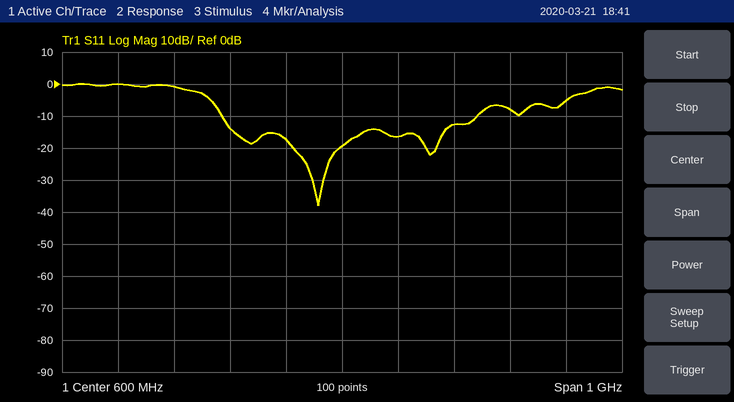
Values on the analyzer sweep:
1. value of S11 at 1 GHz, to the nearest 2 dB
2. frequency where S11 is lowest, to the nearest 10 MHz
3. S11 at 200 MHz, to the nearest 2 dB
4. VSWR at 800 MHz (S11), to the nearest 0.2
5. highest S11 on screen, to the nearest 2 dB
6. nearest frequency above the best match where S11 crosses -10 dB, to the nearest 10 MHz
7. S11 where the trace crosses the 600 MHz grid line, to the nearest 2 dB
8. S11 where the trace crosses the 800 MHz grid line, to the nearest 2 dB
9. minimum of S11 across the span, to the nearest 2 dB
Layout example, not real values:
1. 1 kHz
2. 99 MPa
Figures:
1. -6 dB
2. 560 MHz
3. 0 dB
4. 1.6
5. 0 dB
6. 840 MHz
7. -20 dB
8. -12 dB
9. -38 dB
